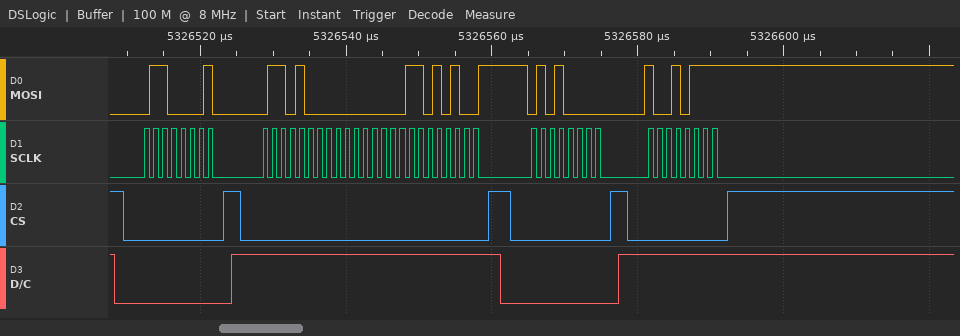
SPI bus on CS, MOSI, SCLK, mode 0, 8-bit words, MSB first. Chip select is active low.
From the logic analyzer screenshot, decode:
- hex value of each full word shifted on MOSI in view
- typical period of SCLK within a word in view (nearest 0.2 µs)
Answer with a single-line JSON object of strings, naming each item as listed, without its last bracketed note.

{"hex value of each full word shifted on MOSI in view": "61, 68, 00, D4, 50, 97", "typical period of SCLK within a word in view": "1.2 µs"}
